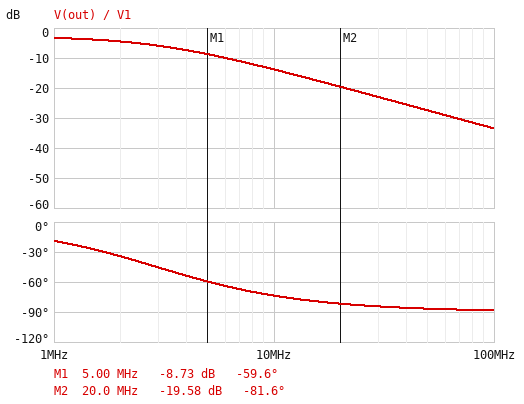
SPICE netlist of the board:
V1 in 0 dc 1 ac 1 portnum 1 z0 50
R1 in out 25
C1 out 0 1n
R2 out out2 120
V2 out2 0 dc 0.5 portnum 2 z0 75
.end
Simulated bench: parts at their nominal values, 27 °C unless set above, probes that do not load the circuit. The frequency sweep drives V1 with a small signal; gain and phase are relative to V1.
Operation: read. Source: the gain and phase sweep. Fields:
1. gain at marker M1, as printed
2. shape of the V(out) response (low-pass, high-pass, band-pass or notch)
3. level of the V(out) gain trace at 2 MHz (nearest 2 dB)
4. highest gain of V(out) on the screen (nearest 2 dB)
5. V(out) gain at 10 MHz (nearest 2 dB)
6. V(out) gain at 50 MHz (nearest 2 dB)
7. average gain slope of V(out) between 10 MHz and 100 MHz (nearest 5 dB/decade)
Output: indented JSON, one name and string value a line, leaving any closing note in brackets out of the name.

{
  "gain at marker M1, as printed": "-8.73 dB",
  "shape of the V(out) response": "low-pass",
  "level of the V(out) gain trace at 2 MHz": "-4 dB",
  "highest gain of V(out) on the screen": "-4 dB",
  "V(out) gain at 10 MHz": "-14 dB",
  "V(out) gain at 50 MHz": "-28 dB",
  "average gain slope of V(out) between 10 MHz and 100 MHz": "-20 dB/decade"
}
